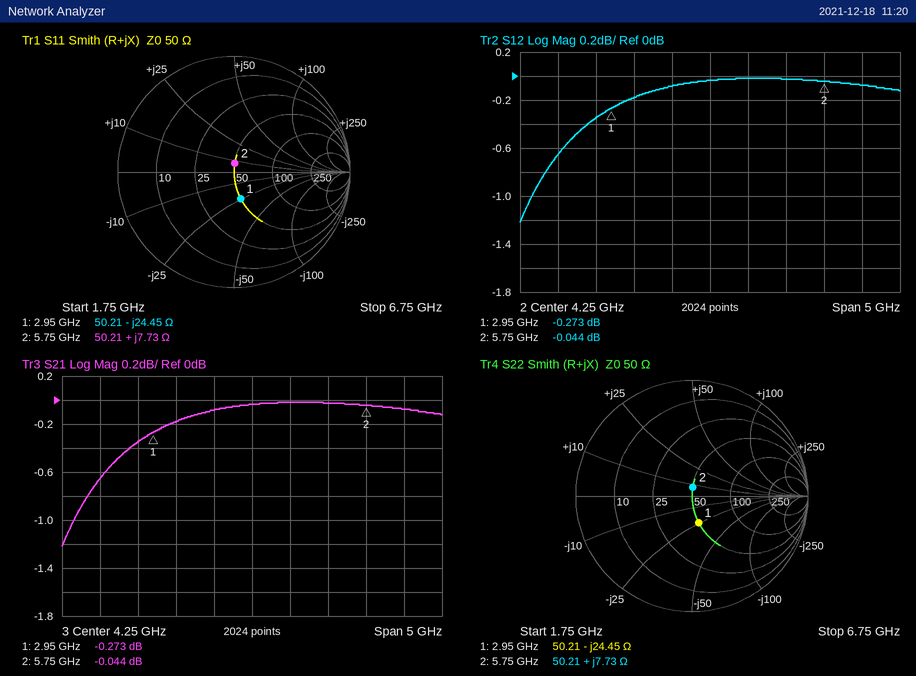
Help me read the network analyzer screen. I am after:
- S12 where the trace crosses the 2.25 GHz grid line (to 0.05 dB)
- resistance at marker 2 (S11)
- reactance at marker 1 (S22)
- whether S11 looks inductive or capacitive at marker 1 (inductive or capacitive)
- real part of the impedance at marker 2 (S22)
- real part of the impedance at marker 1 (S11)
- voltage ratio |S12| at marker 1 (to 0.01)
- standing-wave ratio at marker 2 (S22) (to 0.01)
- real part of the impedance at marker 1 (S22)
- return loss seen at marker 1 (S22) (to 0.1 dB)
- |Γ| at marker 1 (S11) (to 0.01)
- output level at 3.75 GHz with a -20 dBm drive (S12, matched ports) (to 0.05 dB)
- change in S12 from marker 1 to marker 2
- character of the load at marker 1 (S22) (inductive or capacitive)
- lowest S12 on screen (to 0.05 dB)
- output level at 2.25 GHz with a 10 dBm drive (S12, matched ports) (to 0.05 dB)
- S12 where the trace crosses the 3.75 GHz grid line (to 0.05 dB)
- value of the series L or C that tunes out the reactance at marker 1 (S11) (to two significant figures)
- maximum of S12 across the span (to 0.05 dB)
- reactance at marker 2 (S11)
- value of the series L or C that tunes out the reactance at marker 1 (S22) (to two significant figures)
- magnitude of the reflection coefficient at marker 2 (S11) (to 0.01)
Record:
-0.65 dB
50.21 Ω
-24.45 Ω
capacitive
50.21 Ω
50.21 Ω
0.97
1.17
50.21 Ω
12.5 dB
0.24
-20.10 dBm
0.229 dB
capacitive
-1.20 dB
9.35 dBm
-0.10 dB
1.3 nH
0.00 dB
+7.73 Ω
1.3 nH
0.08
